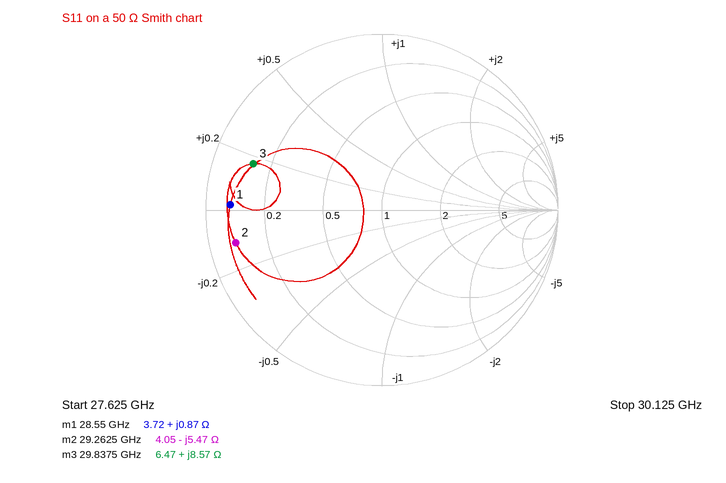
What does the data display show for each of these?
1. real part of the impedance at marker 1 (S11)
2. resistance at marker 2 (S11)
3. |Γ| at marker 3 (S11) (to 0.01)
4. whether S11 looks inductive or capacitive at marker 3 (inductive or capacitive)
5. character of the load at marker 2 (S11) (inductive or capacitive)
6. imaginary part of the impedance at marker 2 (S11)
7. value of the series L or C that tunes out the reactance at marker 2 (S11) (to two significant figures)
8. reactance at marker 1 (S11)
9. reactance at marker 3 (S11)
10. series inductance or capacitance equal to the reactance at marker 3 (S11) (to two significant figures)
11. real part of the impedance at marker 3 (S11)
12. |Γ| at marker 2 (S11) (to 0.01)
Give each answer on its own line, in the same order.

3.72 Ω
4.05 Ω
0.78
inductive
capacitive
-5.47 Ω
30 pH
+0.87 Ω
+8.57 Ω
46 pH
6.47 Ω
0.85
